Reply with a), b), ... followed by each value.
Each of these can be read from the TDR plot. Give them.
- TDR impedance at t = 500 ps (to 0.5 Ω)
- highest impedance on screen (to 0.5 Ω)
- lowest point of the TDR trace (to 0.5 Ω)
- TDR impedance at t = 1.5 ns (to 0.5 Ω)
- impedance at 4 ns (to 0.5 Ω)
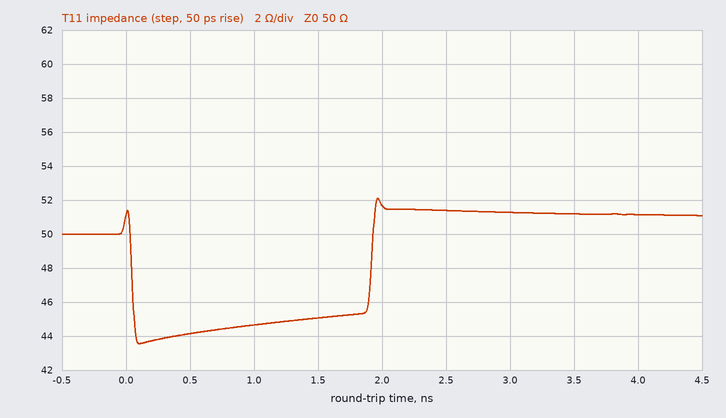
a) 44.0 Ω
b) 52.0 Ω
c) 43.5 Ω
d) 45.0 Ω
e) 51.0 Ω
